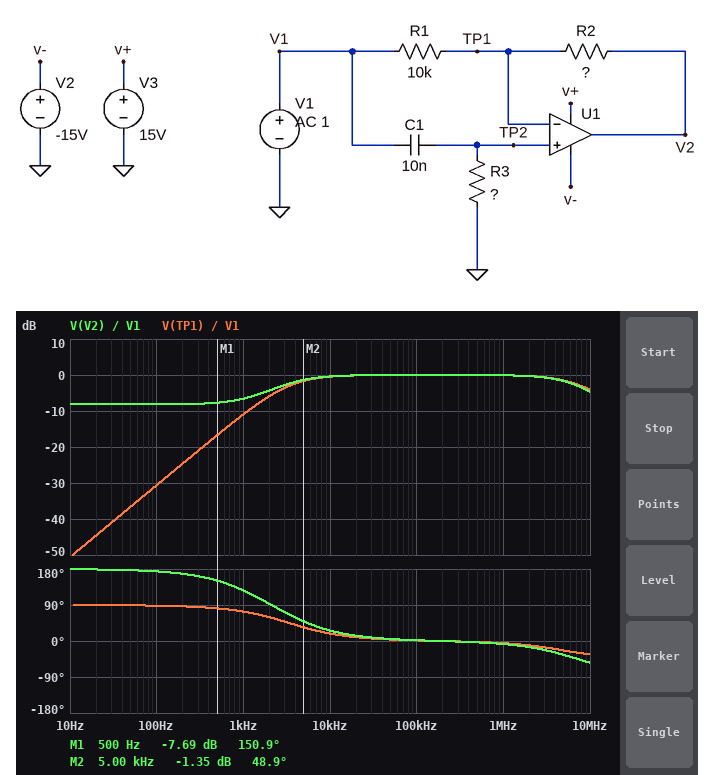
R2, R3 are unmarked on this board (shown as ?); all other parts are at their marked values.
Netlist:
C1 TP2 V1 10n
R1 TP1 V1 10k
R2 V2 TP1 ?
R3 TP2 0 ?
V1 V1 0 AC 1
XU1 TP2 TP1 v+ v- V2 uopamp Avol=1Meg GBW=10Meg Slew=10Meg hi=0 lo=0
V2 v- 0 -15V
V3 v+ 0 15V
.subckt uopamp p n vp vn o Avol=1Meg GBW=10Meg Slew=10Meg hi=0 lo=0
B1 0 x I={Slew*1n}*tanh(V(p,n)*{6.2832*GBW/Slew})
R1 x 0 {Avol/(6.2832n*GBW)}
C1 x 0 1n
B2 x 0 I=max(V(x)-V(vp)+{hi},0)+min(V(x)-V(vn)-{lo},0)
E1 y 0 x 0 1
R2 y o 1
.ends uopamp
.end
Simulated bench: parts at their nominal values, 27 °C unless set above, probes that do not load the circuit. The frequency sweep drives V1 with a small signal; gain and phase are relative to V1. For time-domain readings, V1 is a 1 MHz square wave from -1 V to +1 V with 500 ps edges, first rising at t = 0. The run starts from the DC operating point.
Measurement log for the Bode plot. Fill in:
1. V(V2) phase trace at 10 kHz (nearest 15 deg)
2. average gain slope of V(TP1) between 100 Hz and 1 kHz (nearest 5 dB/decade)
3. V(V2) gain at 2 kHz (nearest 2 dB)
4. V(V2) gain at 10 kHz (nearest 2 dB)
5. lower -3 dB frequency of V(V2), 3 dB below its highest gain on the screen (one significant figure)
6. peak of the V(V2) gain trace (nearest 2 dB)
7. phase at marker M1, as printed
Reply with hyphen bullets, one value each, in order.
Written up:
- 30 deg
- 20 dB/decade
- -4 dB
- 0 dB
- 3 kHz
- 0 dB
- 150.9 deg
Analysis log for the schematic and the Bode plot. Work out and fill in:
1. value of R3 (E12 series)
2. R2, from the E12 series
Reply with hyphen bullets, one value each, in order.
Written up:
- 4.7 kΩ
- 3.9 kΩ
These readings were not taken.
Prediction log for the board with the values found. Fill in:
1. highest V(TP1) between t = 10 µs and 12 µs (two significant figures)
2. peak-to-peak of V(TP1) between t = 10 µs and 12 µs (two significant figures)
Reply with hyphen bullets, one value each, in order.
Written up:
- 1.8 V
- 2.0 V
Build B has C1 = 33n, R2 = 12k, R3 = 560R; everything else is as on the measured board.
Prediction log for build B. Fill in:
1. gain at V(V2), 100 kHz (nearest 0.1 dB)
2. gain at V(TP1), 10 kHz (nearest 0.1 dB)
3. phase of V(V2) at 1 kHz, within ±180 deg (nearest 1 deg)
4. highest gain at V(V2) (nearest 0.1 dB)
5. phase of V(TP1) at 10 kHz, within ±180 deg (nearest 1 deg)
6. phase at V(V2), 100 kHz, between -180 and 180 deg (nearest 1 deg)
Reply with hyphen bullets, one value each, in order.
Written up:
- 0 dB
- -2.4 dB
- 168 deg
- 1.6 dB
- 41 deg
- 10 deg
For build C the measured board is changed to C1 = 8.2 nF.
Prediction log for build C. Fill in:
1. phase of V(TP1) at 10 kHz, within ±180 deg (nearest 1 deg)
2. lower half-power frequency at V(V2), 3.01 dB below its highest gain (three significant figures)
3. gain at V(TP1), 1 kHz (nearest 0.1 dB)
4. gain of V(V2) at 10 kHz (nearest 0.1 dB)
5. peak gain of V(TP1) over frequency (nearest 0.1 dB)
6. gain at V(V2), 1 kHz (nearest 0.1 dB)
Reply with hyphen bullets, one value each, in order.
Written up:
- 22 deg
- 3.44 kHz
- -12.6 dB
- -0.6 dB
- 0 dB
- -7.0 dB
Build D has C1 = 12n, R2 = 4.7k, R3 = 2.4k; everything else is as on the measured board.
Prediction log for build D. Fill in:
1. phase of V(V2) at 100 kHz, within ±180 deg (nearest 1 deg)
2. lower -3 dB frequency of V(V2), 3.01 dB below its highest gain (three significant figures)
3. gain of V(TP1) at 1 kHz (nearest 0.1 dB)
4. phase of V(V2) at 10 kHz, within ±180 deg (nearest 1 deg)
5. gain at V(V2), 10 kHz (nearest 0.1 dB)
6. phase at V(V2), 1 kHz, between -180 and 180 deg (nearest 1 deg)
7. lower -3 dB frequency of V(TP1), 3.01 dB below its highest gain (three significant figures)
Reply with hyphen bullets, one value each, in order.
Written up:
- 4 deg
- 4.12 kHz
- -15.0 dB
- 43 deg
- -0.9 dB
- 149 deg
- 5.52 kHz
